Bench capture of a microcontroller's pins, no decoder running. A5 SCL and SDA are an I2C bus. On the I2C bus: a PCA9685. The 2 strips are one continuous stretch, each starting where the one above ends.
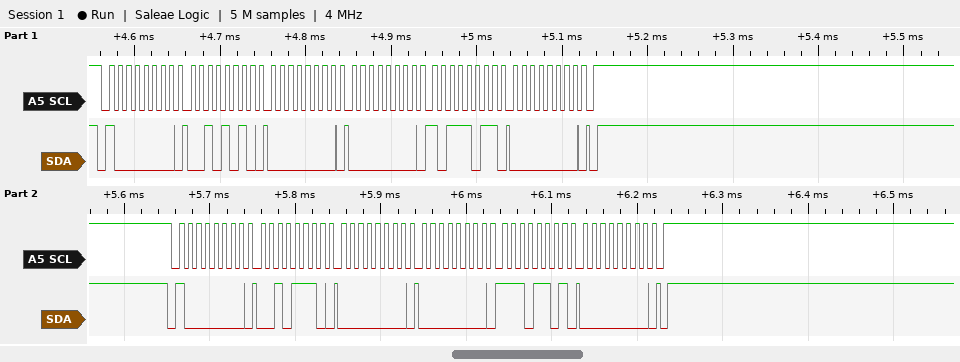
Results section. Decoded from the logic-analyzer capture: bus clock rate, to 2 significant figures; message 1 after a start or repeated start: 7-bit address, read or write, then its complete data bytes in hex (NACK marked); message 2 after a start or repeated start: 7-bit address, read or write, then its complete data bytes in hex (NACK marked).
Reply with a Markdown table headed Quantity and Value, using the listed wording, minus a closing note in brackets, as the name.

| Quantity | Value |
|---|---|
| bus clock rate, to 2 significant figures | 100 kHz |
| message 1 after a start or repeated start: 7-bit address, read or write, then its complete data bytes in hex | 0x40 write: 2A 00 00 BB 00 |
| message 2 after a start or repeated start: 7-bit address, read or write, then its complete data bytes in hex | 0x40 write: 2E 00 00 ED 00 |
